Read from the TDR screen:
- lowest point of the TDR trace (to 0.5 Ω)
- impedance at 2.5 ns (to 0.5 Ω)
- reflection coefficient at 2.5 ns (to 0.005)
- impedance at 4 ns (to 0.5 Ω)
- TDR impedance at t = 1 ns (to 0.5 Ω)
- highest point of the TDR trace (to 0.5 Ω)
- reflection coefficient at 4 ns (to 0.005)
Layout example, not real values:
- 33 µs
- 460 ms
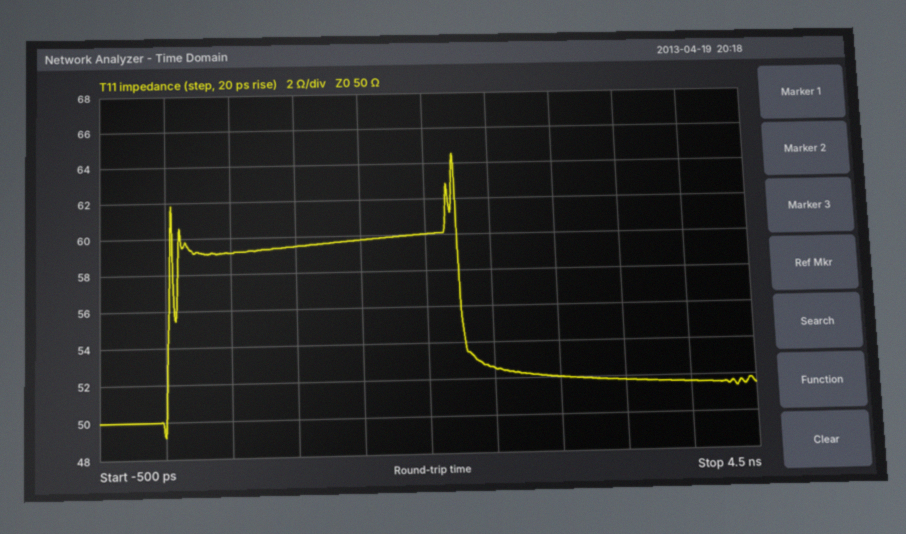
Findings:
- 49.0 Ω
- 52.5 Ω
- +0.025
- 51.5 Ω
- 59.5 Ω
- 64.5 Ω
- +0.015
